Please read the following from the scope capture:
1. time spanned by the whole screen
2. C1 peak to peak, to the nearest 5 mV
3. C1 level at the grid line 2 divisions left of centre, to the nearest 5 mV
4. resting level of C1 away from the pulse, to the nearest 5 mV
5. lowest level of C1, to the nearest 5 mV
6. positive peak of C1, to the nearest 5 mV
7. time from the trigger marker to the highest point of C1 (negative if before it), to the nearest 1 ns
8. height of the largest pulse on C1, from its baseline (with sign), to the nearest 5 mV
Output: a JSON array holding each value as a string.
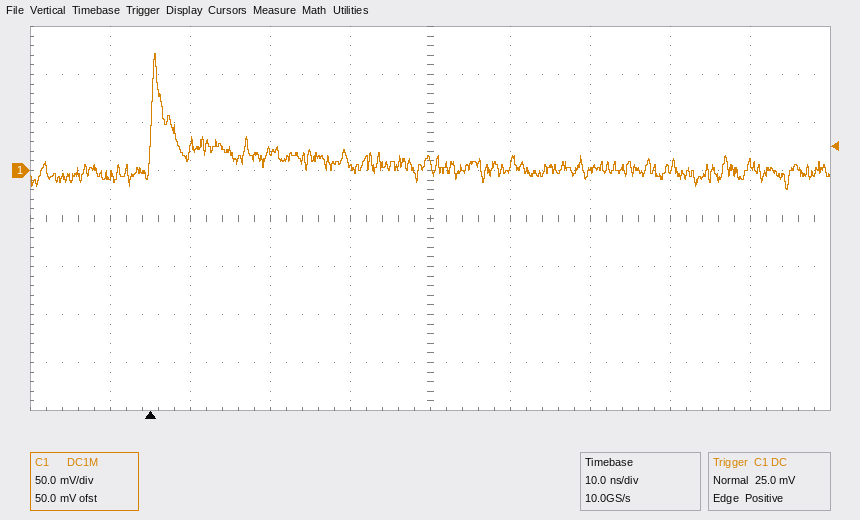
["100 ns", "140 mV", "20 mV", "0 mV", "-20 mV", "120 mV", "+1 ns", "+120 mV"]
